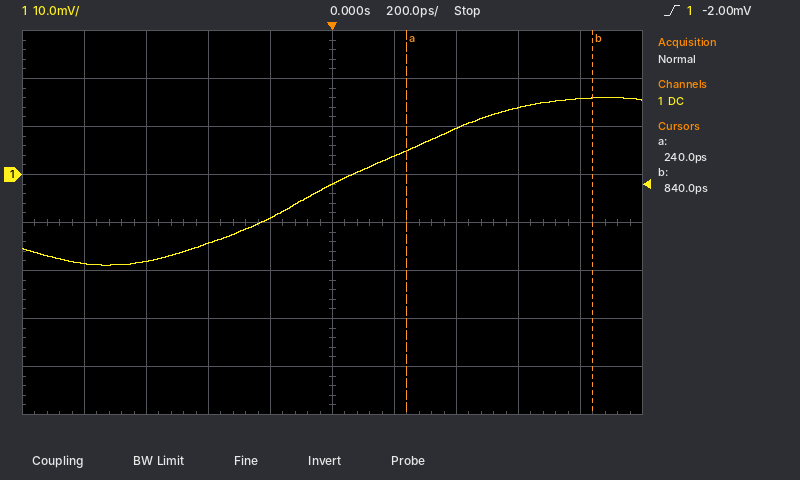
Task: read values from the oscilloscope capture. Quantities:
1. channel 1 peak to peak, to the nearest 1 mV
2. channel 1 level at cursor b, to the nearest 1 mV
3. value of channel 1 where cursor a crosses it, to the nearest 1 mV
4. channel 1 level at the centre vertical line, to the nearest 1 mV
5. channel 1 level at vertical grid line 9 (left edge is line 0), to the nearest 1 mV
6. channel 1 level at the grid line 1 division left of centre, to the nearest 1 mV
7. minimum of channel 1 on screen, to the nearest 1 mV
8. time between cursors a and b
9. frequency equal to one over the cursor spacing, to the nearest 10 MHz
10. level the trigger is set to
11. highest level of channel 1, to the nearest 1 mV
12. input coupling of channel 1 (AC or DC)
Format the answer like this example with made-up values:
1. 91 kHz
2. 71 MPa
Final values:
1. 35 mV
2. 16 mV
3. 5 mV
4. -2 mV
5. 16 mV
6. -9 mV
7. -19 mV
8. 600 ps
9. 1.67 GHz
10. -2.00 mV
11. 16 mV
12. DC
